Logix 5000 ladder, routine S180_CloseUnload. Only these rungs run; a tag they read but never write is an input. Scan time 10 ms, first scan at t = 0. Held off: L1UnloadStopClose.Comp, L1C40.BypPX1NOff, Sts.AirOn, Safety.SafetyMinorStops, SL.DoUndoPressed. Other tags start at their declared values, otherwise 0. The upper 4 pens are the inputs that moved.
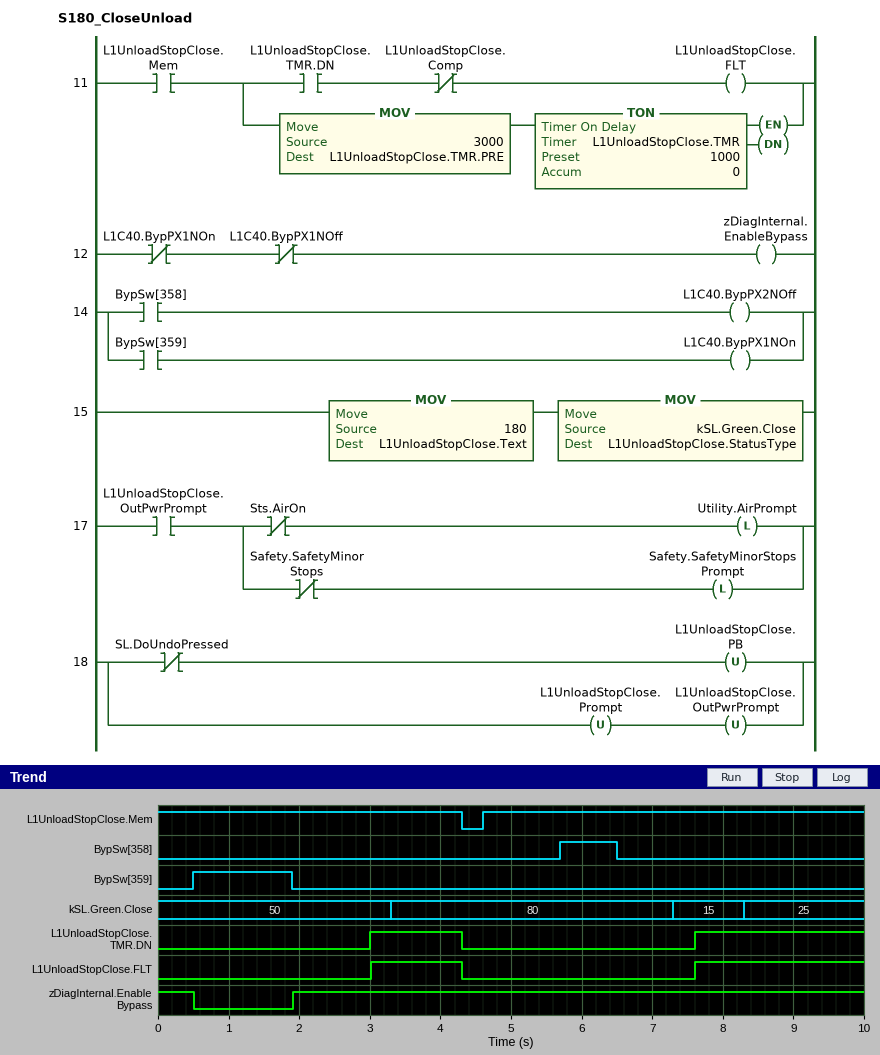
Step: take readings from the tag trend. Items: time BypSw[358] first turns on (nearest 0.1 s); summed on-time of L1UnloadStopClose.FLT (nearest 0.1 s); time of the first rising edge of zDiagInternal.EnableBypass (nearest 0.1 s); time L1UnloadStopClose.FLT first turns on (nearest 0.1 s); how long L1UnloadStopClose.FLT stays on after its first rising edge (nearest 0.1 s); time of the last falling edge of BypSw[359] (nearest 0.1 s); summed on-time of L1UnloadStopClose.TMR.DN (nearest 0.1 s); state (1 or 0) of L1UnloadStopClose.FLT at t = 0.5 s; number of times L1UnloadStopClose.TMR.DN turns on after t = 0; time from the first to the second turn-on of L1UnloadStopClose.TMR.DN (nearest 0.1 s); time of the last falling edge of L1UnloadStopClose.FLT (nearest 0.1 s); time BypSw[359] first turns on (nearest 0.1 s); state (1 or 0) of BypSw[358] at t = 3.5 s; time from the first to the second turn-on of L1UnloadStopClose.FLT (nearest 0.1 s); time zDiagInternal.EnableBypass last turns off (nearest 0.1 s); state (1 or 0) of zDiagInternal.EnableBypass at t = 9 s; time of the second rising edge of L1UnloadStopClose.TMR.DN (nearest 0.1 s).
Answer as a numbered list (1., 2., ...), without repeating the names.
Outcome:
1. 5.7 s
2. 3.7 s
3. 1.9 s
4. 3.0 s
5. 1.3 s
6. 1.9 s
7. 3.7 s
8. 0
9. 2
10. 4.6 s
11. 4.3 s
12. 0.5 s
13. 0
14. 4.6 s
15. 0.5 s
16. 1
17. 7.6 s
